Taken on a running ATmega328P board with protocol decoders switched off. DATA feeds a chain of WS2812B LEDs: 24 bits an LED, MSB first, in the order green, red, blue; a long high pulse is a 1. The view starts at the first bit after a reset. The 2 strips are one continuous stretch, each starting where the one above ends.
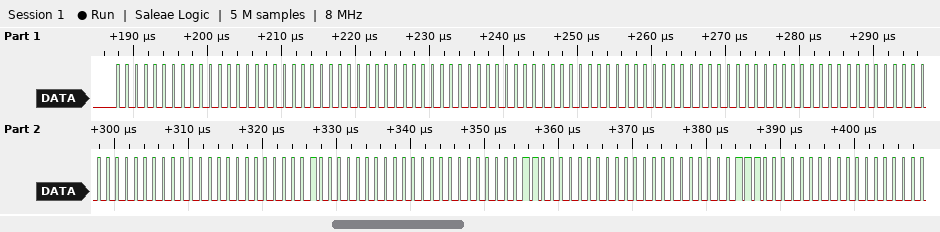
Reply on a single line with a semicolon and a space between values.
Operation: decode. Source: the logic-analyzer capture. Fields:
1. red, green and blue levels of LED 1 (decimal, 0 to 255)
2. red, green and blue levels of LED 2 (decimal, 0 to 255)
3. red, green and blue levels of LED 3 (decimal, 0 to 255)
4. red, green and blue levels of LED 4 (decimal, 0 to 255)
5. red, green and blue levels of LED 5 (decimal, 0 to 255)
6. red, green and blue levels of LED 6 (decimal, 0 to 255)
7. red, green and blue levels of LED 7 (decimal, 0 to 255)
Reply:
0, 0, 0; 0, 0, 0; 0, 0, 0; 0, 0, 0; 1, 0, 0; 3, 0, 0; 7, 0, 0
